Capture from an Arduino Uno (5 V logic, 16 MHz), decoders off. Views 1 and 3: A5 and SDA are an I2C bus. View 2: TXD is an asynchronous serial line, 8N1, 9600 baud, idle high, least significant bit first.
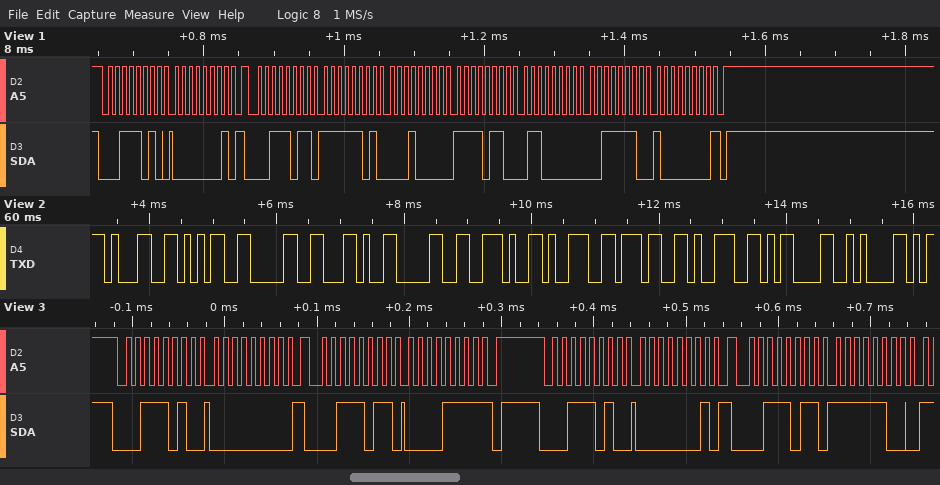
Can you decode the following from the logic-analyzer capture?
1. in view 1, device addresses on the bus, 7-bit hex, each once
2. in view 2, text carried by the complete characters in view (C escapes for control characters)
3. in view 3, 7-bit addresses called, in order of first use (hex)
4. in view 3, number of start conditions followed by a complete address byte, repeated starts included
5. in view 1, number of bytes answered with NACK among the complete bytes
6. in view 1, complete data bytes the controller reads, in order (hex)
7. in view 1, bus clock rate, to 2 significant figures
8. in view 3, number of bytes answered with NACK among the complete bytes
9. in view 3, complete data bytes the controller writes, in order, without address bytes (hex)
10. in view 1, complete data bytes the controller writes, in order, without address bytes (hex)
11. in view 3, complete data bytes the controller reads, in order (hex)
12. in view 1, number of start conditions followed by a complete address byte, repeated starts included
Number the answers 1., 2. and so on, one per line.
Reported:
1. 0x1D
2. "150,0.979\r\n"
3. 0x1D
4. 4
5. 1
6. FD 10 F6 60 3E 80
7. 100 kHz
8. 1
9. 00 01
10. 01
11. 0F FC
12. 2
